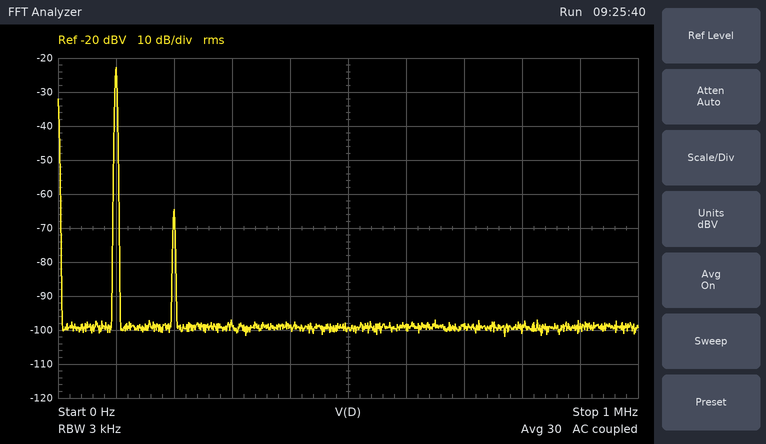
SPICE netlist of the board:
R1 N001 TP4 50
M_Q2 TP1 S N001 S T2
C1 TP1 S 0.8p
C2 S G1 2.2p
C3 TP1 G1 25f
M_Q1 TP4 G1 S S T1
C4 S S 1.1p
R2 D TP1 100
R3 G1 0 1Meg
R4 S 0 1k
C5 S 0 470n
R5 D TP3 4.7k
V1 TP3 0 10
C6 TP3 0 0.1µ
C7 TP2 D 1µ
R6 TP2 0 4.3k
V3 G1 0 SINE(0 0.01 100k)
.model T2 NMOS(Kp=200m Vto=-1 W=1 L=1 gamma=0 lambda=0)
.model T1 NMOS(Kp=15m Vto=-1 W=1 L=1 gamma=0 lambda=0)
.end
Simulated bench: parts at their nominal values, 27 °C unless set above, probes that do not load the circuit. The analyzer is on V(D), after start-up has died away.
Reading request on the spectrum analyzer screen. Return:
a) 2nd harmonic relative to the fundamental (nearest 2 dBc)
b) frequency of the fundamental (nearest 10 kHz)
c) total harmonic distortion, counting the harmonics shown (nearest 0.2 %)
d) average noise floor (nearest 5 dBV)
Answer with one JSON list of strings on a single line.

["-42 dBc", "100 kHz", "0.8 %", "-100 dBV"]
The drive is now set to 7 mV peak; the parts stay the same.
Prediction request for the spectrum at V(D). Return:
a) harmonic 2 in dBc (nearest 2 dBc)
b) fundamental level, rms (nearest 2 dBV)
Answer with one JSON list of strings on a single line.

["-44 dBc", "-26 dBV"]
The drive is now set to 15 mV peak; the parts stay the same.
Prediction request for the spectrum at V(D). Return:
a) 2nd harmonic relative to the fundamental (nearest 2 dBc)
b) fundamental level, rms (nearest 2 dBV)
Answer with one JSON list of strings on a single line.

["-38 dBc", "-20 dBV"]
